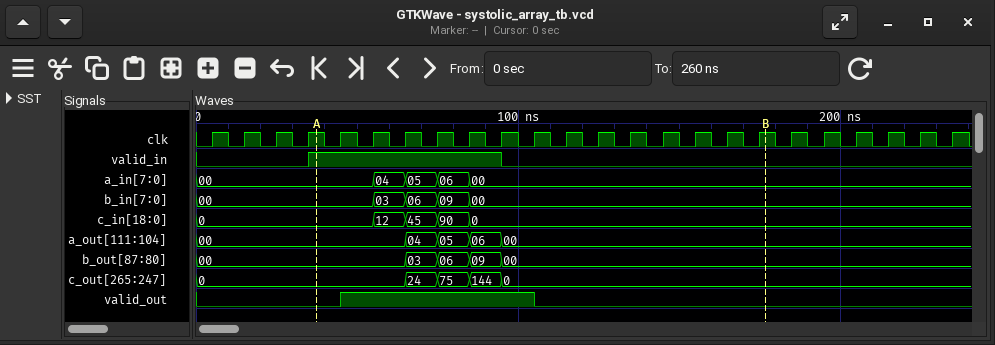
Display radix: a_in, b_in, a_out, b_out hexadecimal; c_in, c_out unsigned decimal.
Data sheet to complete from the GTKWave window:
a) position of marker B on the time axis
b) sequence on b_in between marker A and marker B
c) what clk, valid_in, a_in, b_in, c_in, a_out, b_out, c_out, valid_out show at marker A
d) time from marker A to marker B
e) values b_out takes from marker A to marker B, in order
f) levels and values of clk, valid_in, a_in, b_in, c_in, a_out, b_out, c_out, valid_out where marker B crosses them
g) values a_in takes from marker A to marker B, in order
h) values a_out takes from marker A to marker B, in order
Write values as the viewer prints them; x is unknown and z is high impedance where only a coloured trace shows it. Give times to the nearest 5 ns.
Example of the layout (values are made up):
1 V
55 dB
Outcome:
175 ns
00, 03, 06, 09, 00
clk=1, valid_in=1, a_in=00, b_in=00, c_in=0, a_out=00, b_out=00, c_out=0, valid_out=0
140 ns
00, 03, 06, 09, 00
clk=1, valid_in=0, a_in=00, b_in=00, c_in=0, a_out=00, b_out=00, c_out=0, valid_out=0
00, 04, 05, 06, 00
00, 04, 05, 06, 00
